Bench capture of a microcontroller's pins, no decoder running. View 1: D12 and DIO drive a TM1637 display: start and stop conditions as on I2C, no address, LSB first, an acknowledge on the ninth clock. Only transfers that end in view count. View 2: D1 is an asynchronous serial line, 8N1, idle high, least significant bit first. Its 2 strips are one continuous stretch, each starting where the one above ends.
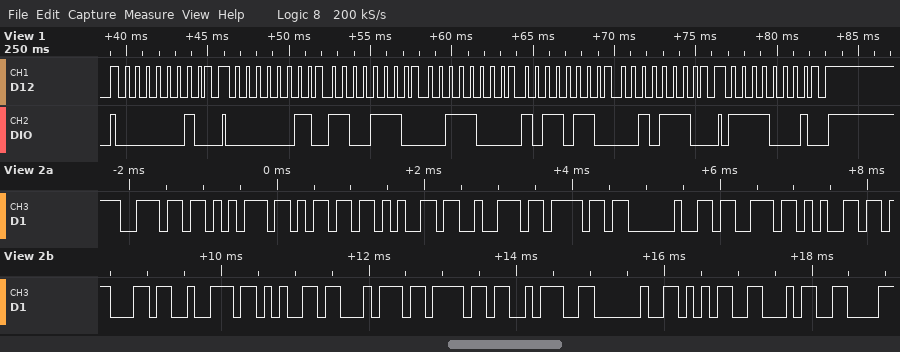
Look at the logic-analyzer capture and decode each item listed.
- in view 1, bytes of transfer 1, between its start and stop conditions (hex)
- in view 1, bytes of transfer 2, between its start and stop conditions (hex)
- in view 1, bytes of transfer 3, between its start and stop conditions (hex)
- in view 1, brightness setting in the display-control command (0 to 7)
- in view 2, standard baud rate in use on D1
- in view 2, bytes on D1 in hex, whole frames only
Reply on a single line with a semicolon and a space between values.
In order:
40; C0 73 1C 6D 74; 8F; 7; 9600 baud; 6E 75 6D 65 72 6F 20 73 65 63 72 65 74 6F 3A 20 35 34
